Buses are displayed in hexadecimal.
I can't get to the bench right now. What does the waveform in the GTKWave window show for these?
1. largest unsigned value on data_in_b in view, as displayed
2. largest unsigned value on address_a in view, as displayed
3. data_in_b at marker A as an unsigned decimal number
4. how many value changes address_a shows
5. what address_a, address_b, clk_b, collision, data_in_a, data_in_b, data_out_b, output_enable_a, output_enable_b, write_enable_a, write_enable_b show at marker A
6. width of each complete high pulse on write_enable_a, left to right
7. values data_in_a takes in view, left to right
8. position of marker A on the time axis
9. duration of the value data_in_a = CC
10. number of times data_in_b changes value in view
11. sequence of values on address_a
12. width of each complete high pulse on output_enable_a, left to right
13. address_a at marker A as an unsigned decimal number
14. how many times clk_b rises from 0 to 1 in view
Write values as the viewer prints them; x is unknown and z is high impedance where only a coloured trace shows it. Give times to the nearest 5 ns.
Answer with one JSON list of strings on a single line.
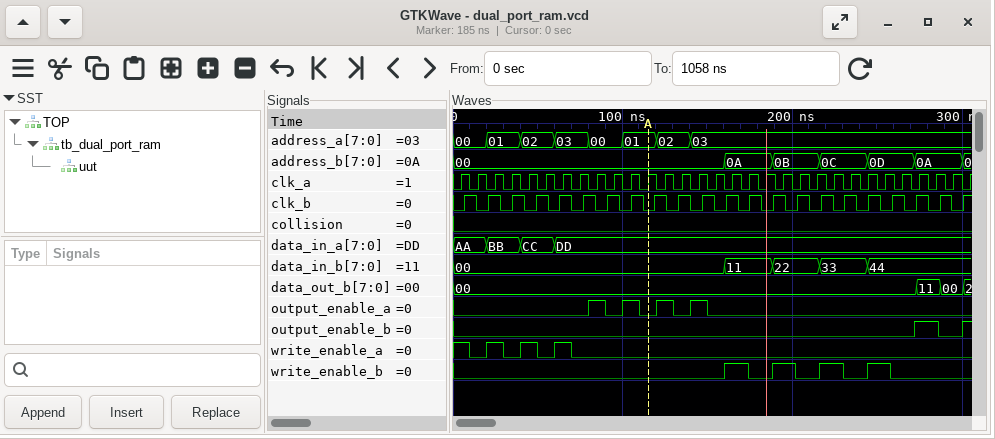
["44", "03", "0", "7", "address_a=01, address_b=00, clk_b=0, collision=0, data_in_a=DD, data_in_b=00, data_out_b=00, output_enable_a=0, output_enable_b=0, write_enable_a=0, write_enable_b=0", "10 ns, 10 ns, 10 ns", "AA, BB, CC, DD", "115 ns", "20 ns", "4", "00, 01, 02, 03, 00, 01, 02, 03", "10 ns, 10 ns, 10 ns, 10 ns", "1", "22"]
